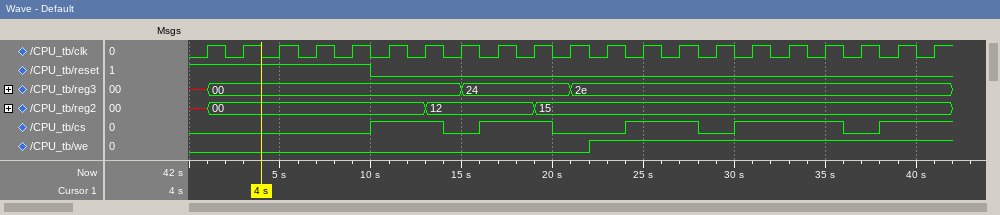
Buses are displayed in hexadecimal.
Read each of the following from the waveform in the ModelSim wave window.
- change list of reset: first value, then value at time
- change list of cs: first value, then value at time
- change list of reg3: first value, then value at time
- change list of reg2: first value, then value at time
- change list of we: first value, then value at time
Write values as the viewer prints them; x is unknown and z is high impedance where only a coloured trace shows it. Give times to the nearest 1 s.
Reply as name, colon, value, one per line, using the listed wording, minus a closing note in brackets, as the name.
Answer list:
change list of reset: first value, then value at time: 1, 0 at 10 s
change list of cs: first value, then value at time: 0, 1 at 10 s, 0 at 14 s, 1 at 16 s, 0 at 20 s, 1 at 24 s, 0 at 28 s, 1 at 30 s, 0 at 36 s, 1 at 38 s
change list of reg3: first value, then value at time: x, 00 at 1 s, 24 at 15 s, 2e at 21 s
change list of reg2: first value, then value at time: x, 00 at 1 s, 12 at 13 s, 15 at 19 s
change list of we: first value, then value at time: 0, 1 at 22 s
